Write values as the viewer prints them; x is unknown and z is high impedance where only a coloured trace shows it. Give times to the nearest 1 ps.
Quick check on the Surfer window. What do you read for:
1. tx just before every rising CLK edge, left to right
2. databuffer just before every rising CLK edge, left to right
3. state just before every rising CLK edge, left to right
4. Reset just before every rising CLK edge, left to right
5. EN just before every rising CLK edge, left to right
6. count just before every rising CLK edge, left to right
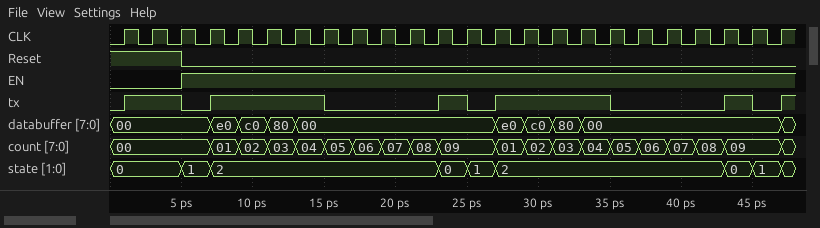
0 1 1 0 1 1 1 1 0 0 0 0 1 0 1 1 1 1 0 0 0 0 1 0
00, 00, 00, 00, e0, c0, 80, 00, 00, 00, 00, 00, 00, 00, e0, c0, 80, 00, 00, 00, 00, 00, 00, 00
0, 0, 0, 1, 2, 2, 2, 2, 2, 2, 2, 2, 0, 1, 2, 2, 2, 2, 2, 2, 2, 2, 0, 1
1 1 1 0 0 0 0 0 0 0 0 0 0 0 0 0 0 0 0 0 0 0 0 0
0 0 0 1 1 1 1 1 1 1 1 1 1 1 1 1 1 1 1 1 1 1 1 1
00, 00, 00, 00, 01, 02, 03, 04, 05, 06, 07, 08, 09, 09, 01, 02, 03, 04, 05, 06, 07, 08, 09, 09
